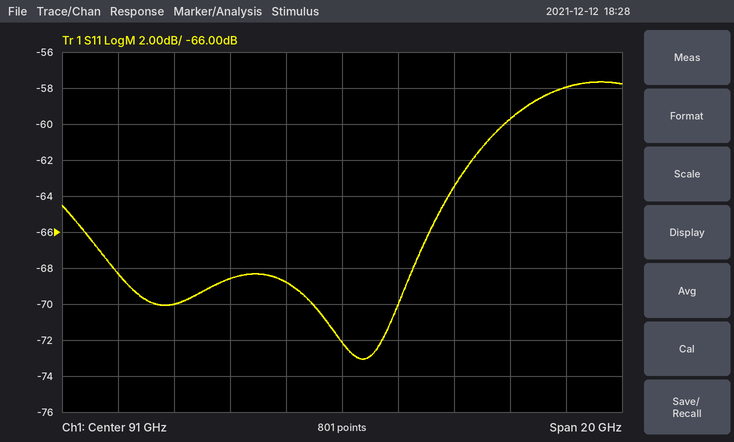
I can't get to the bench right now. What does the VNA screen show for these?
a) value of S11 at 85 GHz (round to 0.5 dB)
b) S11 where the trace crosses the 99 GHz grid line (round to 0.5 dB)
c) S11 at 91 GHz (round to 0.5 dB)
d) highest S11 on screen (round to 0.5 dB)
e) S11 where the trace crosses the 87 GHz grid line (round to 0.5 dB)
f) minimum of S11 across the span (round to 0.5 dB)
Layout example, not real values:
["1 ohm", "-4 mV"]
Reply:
["-70.0 dB", "-58.0 dB", "-72.0 dB", "-57.5 dB", "-68.5 dB", "-73.0 dB"]
